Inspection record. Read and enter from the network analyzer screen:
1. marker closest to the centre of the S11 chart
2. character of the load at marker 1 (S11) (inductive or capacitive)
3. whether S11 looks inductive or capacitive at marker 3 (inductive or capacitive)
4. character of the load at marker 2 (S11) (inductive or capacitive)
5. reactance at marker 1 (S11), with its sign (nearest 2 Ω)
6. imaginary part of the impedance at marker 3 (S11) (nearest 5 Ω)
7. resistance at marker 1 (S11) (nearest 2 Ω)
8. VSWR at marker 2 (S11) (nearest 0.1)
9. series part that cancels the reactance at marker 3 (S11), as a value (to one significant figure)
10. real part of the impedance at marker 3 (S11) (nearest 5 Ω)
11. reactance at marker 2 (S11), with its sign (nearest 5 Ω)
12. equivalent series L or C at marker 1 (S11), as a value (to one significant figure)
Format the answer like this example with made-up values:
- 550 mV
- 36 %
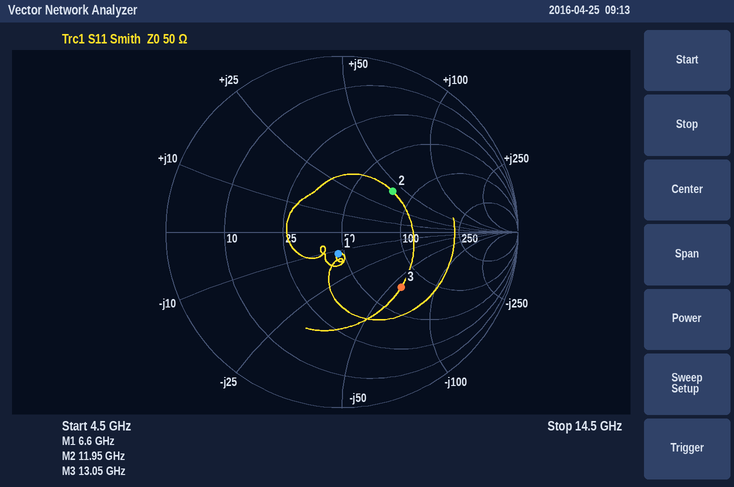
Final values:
- marker 1
- capacitive
- capacitive
- inductive
- -12 Ω
- -60 Ω
- 46 Ω
- 2.2
- 700 pH
- 75 Ω
- +40 Ω
- 2 pF
